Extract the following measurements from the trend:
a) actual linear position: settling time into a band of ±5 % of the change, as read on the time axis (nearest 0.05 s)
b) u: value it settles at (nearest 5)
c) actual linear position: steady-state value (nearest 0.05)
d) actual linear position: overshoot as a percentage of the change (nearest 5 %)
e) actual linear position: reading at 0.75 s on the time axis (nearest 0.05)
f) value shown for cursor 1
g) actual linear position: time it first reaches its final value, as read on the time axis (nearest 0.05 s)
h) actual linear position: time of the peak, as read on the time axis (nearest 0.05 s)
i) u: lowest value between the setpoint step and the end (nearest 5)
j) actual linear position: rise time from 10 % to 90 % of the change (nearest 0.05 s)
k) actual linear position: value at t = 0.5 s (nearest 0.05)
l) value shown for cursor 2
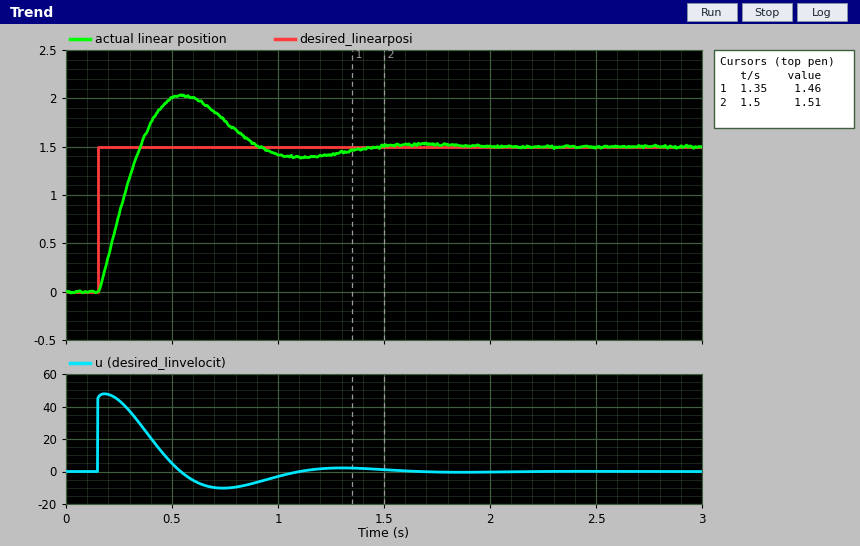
1.25 s
0
1.50
35 %
1.75
1.46
0.35 s
0.55 s
-10
0.15 s
2.00
1.51
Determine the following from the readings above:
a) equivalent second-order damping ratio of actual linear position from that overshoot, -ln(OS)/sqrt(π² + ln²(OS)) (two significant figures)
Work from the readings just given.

0.32
